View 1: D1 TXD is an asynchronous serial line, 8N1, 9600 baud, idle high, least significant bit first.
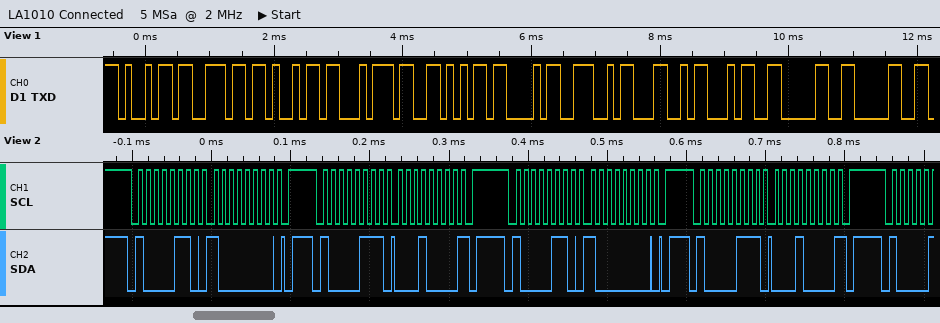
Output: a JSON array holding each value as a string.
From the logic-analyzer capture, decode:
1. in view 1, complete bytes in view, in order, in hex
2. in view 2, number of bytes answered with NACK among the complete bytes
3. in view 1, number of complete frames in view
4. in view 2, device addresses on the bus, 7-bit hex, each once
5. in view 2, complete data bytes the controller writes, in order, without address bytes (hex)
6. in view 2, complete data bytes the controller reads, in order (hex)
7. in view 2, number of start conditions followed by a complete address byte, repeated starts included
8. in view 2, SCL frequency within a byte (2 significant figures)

["69 6E 69 74 56 43 4E 4C 34 30 30", "2", "11", "0x43", "80 80", "10 10", "4", "100 kHz"]
